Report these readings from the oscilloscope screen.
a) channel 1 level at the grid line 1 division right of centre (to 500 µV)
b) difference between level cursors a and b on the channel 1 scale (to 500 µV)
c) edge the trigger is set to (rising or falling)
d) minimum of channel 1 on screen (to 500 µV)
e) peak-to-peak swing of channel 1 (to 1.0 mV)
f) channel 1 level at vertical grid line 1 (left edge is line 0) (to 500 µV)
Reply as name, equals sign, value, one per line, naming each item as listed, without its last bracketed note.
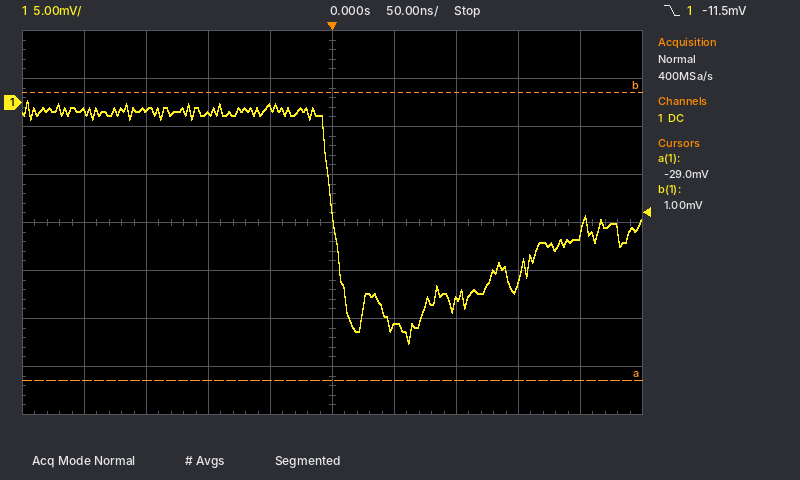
channel 1 level at the grid line 1 division right of centre = -23.5 mV
difference between level cursors a and b on the channel 1 scale = 30.0 mV
edge the trigger is set to = falling
minimum of channel 1 on screen = -25.0 mV
peak-to-peak swing of channel 1 = 25.0 mV
channel 1 level at vertical grid line 1 (left edge is line 0) = -1.0 mV
